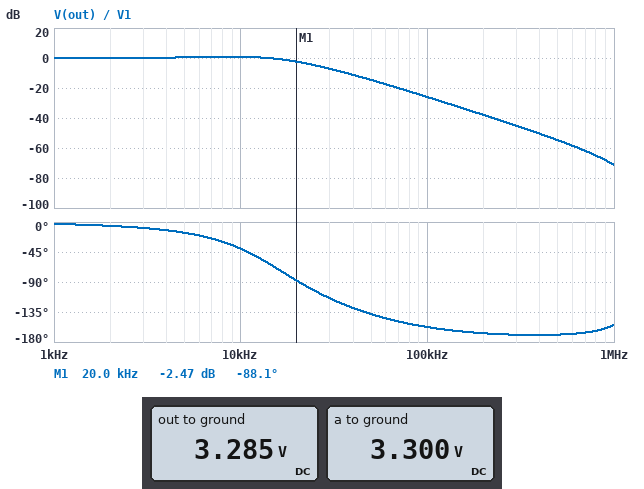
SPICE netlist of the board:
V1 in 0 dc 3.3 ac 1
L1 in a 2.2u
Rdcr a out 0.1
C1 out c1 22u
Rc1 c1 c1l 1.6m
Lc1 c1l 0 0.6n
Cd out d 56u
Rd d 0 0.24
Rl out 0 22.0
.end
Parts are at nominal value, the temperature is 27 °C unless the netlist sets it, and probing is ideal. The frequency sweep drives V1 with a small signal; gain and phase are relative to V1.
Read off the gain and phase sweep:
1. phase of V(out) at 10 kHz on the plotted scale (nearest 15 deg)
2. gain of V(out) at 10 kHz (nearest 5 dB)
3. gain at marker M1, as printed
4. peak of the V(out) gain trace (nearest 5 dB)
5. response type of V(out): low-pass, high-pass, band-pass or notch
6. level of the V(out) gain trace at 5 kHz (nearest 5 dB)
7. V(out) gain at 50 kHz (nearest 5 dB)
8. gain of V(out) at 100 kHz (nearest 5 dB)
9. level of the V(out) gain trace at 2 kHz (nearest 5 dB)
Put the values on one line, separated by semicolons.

-45 deg; 0 dB; -2.47 dB; 0 dB; low-pass; 0 dB; -15 dB; -25 dB; 0 dB
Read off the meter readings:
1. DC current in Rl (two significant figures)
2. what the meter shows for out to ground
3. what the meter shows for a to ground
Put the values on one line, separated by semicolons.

150 mA; 3.285 V; 3.300 V
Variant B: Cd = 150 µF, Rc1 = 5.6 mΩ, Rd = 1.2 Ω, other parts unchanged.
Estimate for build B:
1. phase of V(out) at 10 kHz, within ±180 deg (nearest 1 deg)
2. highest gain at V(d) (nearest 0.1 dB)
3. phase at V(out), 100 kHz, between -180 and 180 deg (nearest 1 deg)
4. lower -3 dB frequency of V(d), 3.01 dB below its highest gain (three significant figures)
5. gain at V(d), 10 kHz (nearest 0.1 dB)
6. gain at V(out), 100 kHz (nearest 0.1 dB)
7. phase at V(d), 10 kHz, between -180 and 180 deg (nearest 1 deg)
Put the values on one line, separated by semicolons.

-17 deg; 4.3 dB; -167 deg; 12.1 kHz; 0.6 dB; -25.3 dB; -12 deg
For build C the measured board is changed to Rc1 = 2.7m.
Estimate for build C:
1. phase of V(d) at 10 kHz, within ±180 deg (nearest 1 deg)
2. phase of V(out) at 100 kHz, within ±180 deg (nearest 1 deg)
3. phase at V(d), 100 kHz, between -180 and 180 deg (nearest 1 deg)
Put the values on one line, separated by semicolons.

10 deg; -157 deg; -150 deg
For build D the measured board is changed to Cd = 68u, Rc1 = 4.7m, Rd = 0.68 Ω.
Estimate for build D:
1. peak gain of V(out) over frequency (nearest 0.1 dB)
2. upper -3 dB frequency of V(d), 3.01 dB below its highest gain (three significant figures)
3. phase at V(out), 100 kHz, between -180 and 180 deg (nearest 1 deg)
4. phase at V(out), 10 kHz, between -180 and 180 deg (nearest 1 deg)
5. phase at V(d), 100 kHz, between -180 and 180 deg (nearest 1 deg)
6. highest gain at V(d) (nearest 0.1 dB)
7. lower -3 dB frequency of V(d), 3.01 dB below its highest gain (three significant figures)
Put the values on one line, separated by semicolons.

2.1 dB; 28.4 kHz; -165 deg; -23 deg; -163 deg; 2.0 dB; 6.98 kHz
